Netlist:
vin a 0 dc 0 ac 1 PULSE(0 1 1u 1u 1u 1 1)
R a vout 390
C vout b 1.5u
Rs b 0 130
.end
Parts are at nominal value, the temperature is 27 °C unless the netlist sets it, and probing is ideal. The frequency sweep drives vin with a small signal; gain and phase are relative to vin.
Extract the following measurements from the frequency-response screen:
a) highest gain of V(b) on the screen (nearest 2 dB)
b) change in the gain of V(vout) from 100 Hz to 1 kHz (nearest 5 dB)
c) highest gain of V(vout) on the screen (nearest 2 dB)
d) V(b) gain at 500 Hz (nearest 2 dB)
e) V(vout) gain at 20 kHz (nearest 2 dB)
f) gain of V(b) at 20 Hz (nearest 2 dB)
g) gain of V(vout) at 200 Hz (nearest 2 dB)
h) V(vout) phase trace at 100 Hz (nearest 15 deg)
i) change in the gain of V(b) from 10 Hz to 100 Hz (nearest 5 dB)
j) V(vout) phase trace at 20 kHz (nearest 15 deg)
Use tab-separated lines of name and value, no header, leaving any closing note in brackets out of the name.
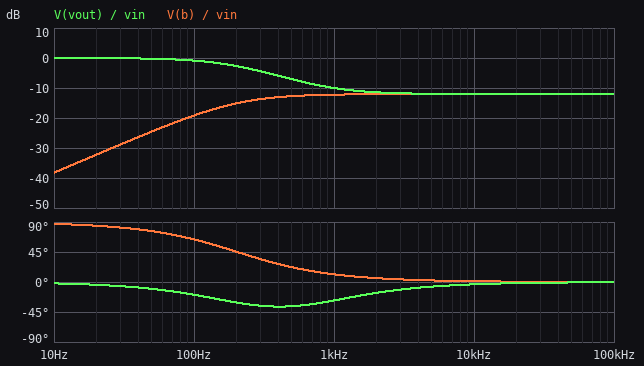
highest gain of V(b) on the screen	-12 dB
change in the gain of V(vout) from 100 Hz to 1 kHz	-10 dB
highest gain of V(vout) on the screen	0 dB
V(b) gain at 500 Hz	-12 dB
V(vout) gain at 20 kHz	-12 dB
gain of V(b) at 20 Hz	-32 dB
gain of V(vout) at 200 Hz	-2 dB
V(vout) phase trace at 100 Hz	-15 deg
change in the gain of V(b) from 10 Hz to 100 Hz	20 dB
V(vout) phase trace at 20 kHz	0 deg
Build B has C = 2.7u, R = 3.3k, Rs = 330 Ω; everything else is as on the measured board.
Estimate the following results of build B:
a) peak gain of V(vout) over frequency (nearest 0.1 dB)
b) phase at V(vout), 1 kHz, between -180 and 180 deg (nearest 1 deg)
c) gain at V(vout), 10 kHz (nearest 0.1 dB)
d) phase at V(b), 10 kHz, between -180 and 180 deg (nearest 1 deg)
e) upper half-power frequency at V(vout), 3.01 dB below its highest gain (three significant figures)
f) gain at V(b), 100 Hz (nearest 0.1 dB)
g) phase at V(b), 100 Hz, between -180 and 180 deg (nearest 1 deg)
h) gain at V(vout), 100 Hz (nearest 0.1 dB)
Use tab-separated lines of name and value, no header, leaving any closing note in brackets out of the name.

peak gain of V(vout) over frequency	0 dB
phase at V(vout), 1 kHz, between -180 and 180 deg	-9 deg
gain at V(vout), 10 kHz	-20.8 dB
phase at V(b), 10 kHz, between -180 and 180 deg	0 deg
upper half-power frequency at V(vout), 3.01 dB below its highest gain	16.4 Hz
gain at V(b), 100 Hz	-20.9 dB
phase at V(b), 100 Hz, between -180 and 180 deg	9 deg
gain at V(vout), 100 Hz	-14.7 dB
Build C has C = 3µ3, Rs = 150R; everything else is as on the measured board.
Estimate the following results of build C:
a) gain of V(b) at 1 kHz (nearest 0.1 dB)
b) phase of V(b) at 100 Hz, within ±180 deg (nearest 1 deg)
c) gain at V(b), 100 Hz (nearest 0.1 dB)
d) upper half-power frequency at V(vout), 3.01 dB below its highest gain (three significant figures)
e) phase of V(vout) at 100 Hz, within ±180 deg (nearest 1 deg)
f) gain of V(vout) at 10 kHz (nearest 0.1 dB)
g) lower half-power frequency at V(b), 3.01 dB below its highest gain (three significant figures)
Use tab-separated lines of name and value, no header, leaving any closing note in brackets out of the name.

gain of V(b) at 1 kHz	-11.2 dB
phase of V(b) at 100 Hz, within ±180 deg	42 deg
gain at V(b), 100 Hz	-13.7 dB
upper half-power frequency at V(vout), 3.01 dB below its highest gain	97.1 Hz
phase of V(vout) at 100 Hz, within ±180 deg	-31 deg
gain of V(vout) at 10 kHz	-11.1 dB
lower half-power frequency at V(b), 3.01 dB below its highest gain	89.3 Hz
